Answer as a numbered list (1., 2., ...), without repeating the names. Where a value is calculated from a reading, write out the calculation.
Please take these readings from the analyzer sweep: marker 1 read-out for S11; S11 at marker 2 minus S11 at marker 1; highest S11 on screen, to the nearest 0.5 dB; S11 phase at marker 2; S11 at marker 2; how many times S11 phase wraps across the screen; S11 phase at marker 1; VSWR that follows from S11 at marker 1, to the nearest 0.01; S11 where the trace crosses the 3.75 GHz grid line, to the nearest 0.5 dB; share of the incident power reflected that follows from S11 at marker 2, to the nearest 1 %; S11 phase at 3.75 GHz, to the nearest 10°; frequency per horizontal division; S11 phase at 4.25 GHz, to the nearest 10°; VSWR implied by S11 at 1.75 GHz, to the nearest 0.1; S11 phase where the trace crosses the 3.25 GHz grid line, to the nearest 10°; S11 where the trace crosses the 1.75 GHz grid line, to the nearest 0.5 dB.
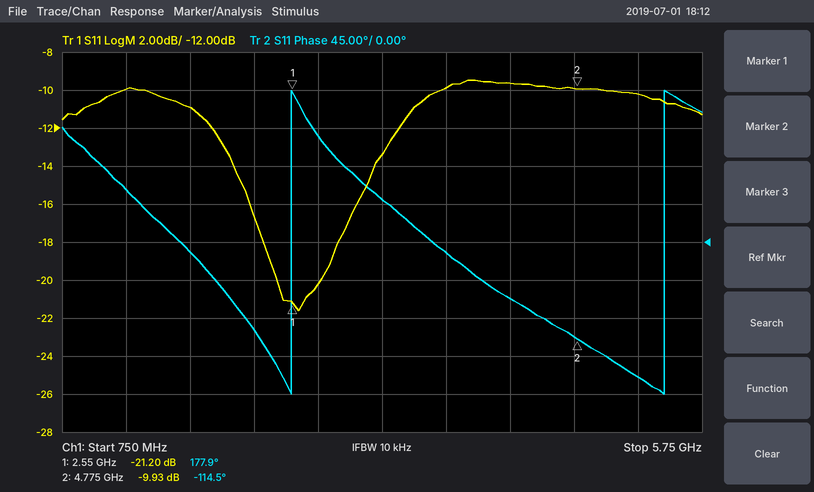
1. -21.20 dB
2. -9.93 − (-21.2) = 11.27 dB
3. -9.5 dB
4. -114.5°
5. -9.93 dB
6. 2
7. 177.9°
8. (1 + 0.0871)/(1 − 0.0871) ≈ 1.19
9. -10.0 dB
10. 10^(-9.93/10) ≈ 10 %
11. -10°
12. 500 MHz
13. -70°
14. |Γ| = 10^(-11/20) = 0.2818; VSWR = (1 + 0.2818)/(1 − 0.2818) ≈ 1.8
15. 50°
16. -11.0 dB
